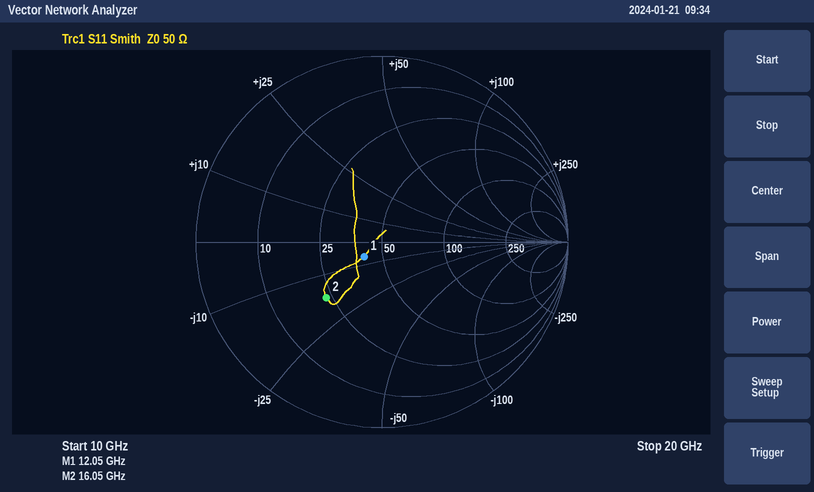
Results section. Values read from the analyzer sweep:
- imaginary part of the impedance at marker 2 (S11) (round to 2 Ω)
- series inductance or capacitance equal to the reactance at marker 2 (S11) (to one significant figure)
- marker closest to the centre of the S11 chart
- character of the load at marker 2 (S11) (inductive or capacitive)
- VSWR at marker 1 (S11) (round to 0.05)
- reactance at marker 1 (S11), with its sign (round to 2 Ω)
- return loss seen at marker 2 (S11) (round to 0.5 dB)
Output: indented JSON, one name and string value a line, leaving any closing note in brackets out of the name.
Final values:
{
  "imaginary part of the impedance at marker 2 (S11)": "-16 Ω",
  "series inductance or capacitance equal to the reactance at marker 2 (S11)": "600 fF",
  "marker closest to the centre of the S11 chart": "marker 1",
  "character of the load at marker 2 (S11)": "capacitive",
  "VSWR at marker 1 (S11)": "1.30",
  "reactance at marker 1 (S11), with its sign": "-6 Ω",
  "return loss seen at marker 2 (S11)": "7.5 dB"
}
